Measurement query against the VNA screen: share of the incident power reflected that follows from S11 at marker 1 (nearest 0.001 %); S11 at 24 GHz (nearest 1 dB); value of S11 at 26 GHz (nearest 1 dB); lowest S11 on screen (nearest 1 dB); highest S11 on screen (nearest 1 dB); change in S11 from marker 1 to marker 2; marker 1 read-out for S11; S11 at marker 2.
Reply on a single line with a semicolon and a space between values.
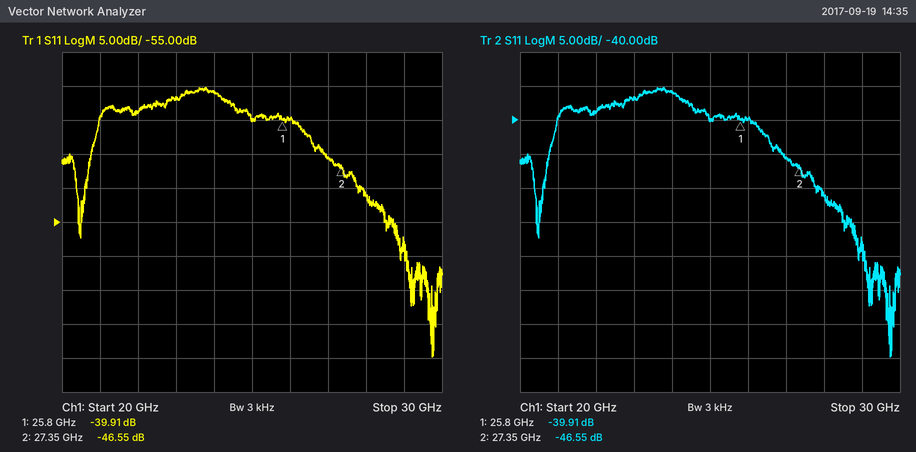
0.010 %; -36 dB; -40 dB; -75 dB; -35 dB; -6.64 dB; -39.91 dB; -46.55 dB
